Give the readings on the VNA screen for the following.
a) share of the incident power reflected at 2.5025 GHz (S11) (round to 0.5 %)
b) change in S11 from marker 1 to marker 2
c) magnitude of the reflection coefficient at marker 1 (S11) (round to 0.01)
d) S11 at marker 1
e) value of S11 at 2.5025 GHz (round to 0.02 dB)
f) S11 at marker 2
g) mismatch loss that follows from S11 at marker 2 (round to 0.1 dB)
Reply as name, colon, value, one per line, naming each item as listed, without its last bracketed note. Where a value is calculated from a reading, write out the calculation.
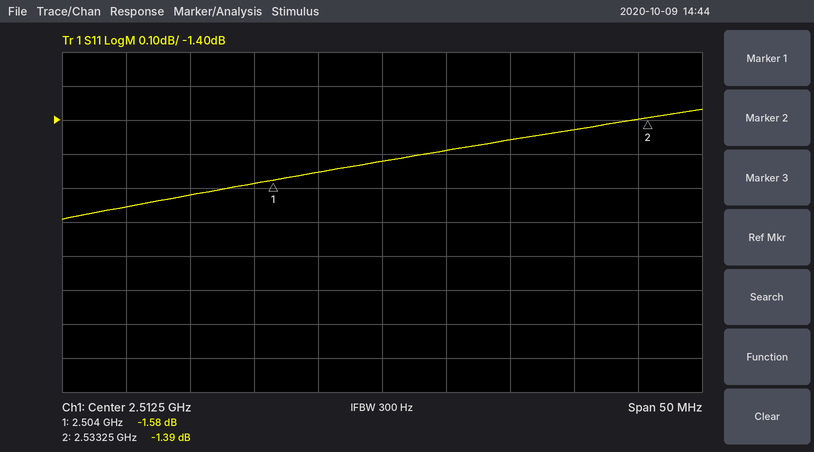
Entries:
share of the incident power reflected at 2.5025 GHz (S11): 10^(-1.58/10) ≈ 69.5 %
change in S11 from marker 1 to marker 2: -1.39 − (-1.58) = 0.19 dB
magnitude of the reflection coefficient at marker 1 (S11): 10^(-1.58/20) ≈ 0.83
S11 at marker 1: -1.58 dB
value of S11 at 2.5025 GHz: -1.58 dB
S11 at marker 2: -1.39 dB
mismatch loss that follows from S11 at marker 2: −10 log10(1 − 10^(-1.39/10)) ≈ 5.6 dB
